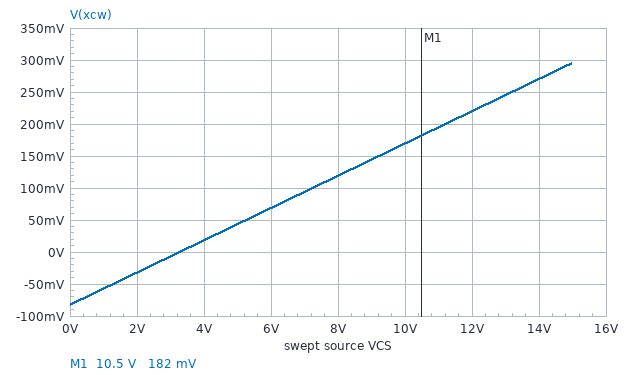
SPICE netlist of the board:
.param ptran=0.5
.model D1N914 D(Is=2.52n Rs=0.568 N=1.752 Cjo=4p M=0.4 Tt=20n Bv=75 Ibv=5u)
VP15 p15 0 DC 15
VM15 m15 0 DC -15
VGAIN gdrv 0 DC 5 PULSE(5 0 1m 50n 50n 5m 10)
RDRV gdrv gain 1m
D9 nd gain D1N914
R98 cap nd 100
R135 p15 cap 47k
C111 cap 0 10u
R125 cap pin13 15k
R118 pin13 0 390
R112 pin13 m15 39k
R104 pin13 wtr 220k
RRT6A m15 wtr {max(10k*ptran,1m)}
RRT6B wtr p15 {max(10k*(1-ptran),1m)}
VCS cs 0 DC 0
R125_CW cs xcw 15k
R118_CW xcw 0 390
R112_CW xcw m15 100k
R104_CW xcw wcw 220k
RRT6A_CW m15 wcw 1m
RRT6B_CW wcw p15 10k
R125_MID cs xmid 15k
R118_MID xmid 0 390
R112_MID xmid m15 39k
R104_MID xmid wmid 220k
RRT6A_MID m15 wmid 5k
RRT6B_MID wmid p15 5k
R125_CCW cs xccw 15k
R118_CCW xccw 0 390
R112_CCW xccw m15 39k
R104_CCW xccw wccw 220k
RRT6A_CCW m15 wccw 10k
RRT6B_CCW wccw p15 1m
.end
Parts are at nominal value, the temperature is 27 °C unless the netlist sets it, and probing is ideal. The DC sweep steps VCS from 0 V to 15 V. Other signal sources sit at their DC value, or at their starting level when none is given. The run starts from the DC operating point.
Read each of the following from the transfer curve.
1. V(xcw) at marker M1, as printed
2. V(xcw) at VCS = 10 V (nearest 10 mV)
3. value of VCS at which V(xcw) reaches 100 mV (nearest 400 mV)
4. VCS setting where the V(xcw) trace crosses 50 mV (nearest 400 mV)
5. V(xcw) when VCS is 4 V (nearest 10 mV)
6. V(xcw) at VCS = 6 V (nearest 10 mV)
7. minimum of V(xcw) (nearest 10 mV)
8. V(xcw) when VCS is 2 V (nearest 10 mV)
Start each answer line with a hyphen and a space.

- 182 mV
- 170 mV
- 7.2 V
- 5.2 V
- 20 mV
- 70 mV
- -80 mV
- -30 mV
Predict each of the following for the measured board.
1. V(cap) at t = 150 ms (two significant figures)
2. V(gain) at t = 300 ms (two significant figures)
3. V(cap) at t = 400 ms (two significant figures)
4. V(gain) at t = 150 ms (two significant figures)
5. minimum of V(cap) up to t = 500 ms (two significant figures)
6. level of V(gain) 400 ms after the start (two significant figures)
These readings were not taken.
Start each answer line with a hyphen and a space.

- 2.7 V
- 5.0 V
- 3.5 V
- 5.0 V
- 630 mV
- 5.0 V
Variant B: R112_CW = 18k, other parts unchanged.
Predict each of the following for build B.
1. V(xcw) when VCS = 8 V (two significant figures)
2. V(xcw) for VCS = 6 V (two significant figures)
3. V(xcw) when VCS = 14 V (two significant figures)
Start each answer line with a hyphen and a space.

- -140 mV
- -190 mV
- 12 mV
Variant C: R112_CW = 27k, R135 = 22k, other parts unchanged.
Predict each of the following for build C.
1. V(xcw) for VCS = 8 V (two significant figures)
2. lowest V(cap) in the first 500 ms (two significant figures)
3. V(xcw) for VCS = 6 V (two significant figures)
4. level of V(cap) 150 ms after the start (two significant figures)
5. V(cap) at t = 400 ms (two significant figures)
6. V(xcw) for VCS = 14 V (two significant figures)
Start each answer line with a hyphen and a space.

- -34 mV
- 700 mV
- -84 mV
- 5.0 V
- 5.5 V
- 120 mV
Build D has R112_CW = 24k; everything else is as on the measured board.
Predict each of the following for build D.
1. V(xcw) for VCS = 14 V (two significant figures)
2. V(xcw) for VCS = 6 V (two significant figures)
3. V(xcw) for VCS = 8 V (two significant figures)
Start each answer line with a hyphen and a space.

- 90 mV
- -110 mV
- -60 mV
